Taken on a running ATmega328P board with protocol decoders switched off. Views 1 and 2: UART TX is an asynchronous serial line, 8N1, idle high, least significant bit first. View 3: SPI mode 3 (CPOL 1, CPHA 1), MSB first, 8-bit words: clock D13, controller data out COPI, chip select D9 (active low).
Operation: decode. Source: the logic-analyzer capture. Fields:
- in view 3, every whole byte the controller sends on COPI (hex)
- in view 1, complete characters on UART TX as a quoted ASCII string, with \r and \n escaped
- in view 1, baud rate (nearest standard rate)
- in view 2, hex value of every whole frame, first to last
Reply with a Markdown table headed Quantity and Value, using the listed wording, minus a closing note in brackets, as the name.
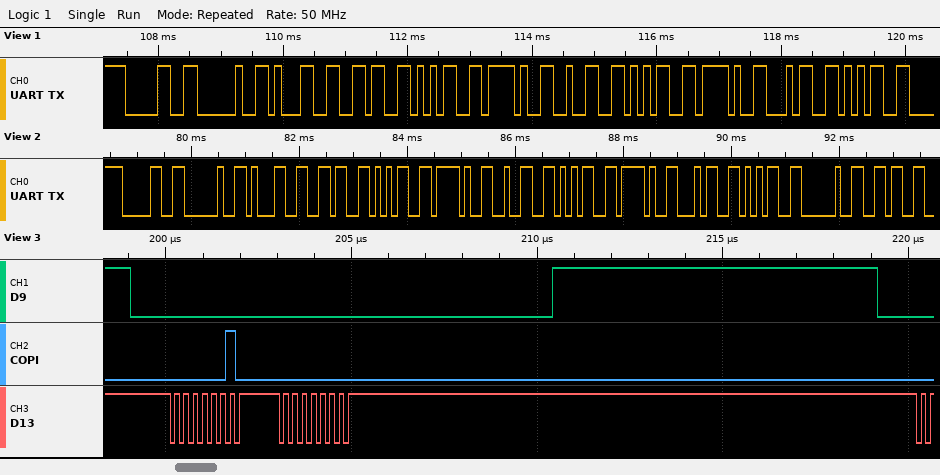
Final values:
| Quantity | Value |
|---|---|
| in view 3, every whole byte the controller sends on COPI | 02 00 |
| in view 1, complete characters on UART TX as a quoted ASCII string, with \r and \n escaped | "0 165/25/45" |
| in view 1, baud rate | 9600 baud |
| in view 2, hex value of every whole frame, first to last | 30 20 31 36 35 2F 32 35 2F 34 35 20 36 |
